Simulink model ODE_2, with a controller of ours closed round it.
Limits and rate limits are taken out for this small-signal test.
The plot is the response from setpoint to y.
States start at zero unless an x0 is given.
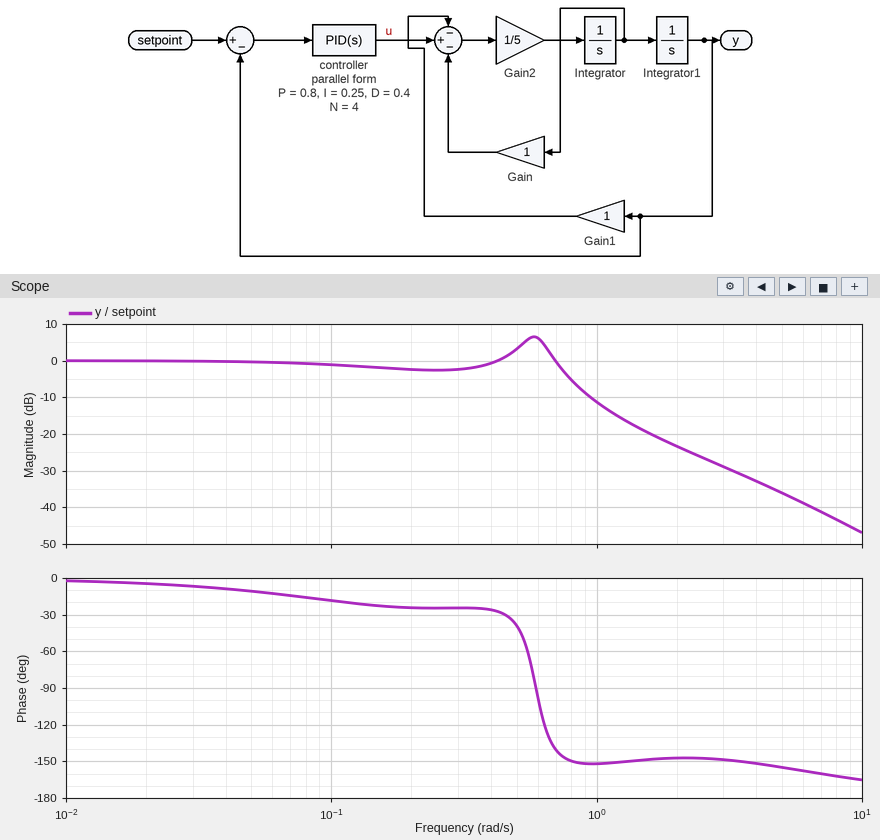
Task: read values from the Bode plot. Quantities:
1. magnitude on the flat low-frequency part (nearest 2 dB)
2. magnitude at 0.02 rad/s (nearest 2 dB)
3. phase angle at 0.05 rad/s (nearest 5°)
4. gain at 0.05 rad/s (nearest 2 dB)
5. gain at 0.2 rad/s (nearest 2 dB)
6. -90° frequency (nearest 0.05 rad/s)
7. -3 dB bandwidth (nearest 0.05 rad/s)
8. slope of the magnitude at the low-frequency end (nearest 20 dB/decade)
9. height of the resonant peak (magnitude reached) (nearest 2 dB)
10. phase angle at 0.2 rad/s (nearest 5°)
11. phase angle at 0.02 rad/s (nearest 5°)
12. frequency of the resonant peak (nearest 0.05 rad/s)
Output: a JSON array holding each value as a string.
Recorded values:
["0 dB", "0 dB", "-10°", "0 dB", "-2 dB", "0.60 rad/s", "0.75 rad/s", "0 dB/decade", "6 dB", "-25°", "-5°", "0.60 rad/s"]
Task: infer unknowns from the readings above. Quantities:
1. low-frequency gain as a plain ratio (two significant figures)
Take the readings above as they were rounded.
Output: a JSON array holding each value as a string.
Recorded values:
["1.0"]
